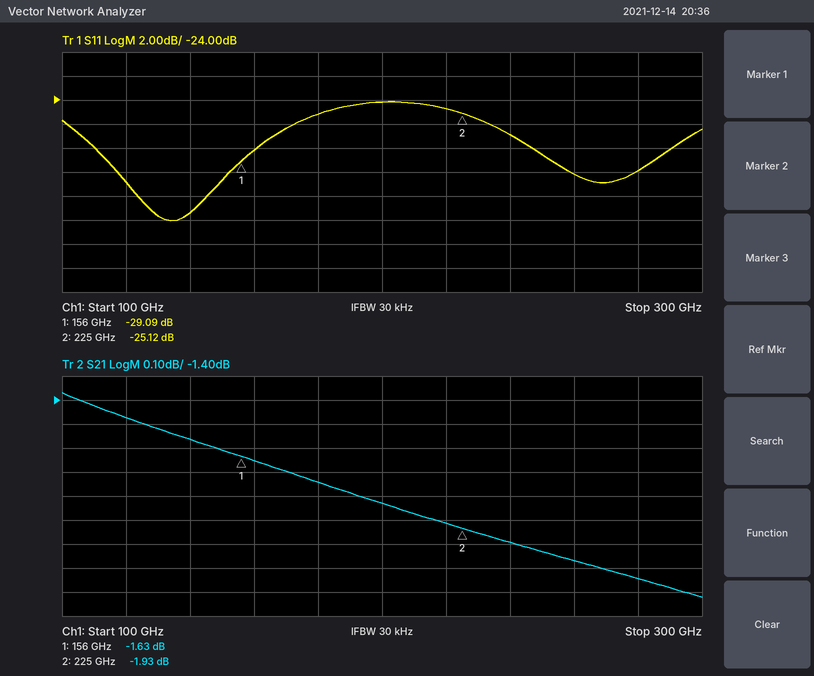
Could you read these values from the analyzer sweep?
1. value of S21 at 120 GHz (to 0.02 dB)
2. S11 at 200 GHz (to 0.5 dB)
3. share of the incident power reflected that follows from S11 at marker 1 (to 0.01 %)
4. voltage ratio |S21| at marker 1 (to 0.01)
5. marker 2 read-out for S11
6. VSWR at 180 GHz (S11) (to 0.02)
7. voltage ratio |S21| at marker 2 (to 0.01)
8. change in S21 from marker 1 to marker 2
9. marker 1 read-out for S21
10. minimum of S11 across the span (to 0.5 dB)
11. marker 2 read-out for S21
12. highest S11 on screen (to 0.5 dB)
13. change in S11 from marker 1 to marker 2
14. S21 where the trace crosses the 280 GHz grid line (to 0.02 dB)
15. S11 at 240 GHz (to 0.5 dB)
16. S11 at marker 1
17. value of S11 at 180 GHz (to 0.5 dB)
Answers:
-1.48 dB
-24.0 dB
0.12 %
0.83
-25.12 dB
1.12
0.80
-0.30 dB
-1.63 dB
-34.0 dB
-1.93 dB
-24.0 dB
3.97 dB
-2.14 dB
-27.0 dB
-29.09 dB
-25.0 dB
